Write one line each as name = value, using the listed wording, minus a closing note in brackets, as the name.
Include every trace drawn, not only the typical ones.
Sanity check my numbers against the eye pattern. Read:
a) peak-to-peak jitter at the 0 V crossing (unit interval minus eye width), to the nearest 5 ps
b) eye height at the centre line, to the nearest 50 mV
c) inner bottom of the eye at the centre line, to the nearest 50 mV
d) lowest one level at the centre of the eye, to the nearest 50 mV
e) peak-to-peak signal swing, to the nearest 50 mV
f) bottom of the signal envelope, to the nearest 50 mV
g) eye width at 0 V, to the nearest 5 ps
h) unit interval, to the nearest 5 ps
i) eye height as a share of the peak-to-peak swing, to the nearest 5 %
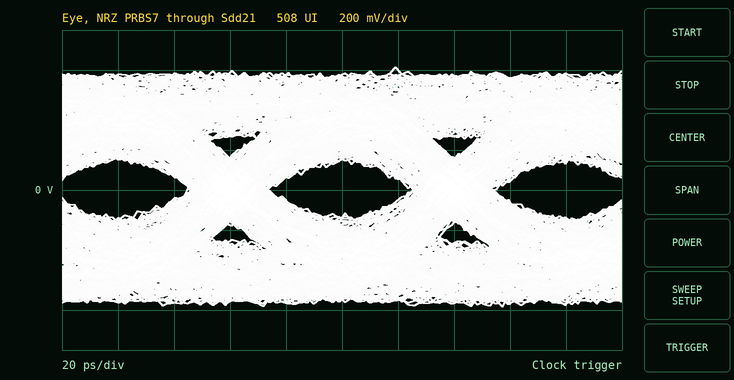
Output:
peak-to-peak jitter at the 0 V crossing (unit interval minus eye width), to the nearest 5 ps = 30 ps
eye height at the centre line, to the nearest 50 mV = 300 mV
inner bottom of the eye at the centre line, to the nearest 50 mV = -150 mV
lowest one level at the centre of the eye, to the nearest 50 mV = 150 mV
peak-to-peak signal swing, to the nearest 50 mV = 1.20 V
bottom of the signal envelope, to the nearest 50 mV = -600 mV
eye width at 0 V, to the nearest 5 ps = 50 ps
unit interval, to the nearest 5 ps = 80 ps
eye height as a share of the peak-to-peak swing, to the nearest 5 % = 25 %
